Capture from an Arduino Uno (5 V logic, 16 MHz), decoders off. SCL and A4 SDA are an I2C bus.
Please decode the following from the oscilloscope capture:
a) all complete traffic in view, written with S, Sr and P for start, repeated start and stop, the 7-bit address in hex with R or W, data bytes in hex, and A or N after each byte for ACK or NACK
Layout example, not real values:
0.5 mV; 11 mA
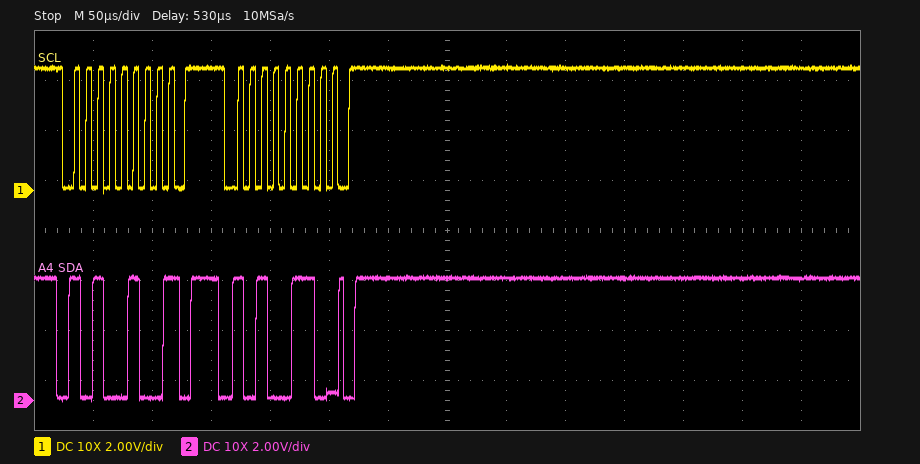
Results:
S 52W N P S 53W A P
